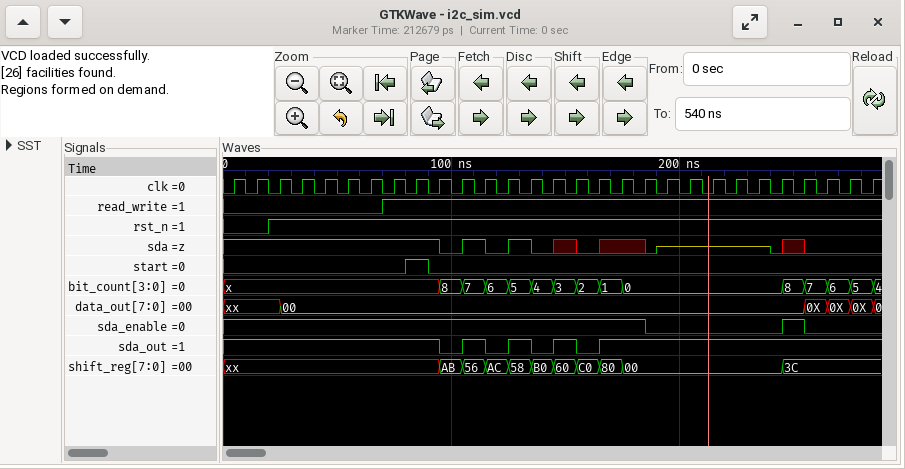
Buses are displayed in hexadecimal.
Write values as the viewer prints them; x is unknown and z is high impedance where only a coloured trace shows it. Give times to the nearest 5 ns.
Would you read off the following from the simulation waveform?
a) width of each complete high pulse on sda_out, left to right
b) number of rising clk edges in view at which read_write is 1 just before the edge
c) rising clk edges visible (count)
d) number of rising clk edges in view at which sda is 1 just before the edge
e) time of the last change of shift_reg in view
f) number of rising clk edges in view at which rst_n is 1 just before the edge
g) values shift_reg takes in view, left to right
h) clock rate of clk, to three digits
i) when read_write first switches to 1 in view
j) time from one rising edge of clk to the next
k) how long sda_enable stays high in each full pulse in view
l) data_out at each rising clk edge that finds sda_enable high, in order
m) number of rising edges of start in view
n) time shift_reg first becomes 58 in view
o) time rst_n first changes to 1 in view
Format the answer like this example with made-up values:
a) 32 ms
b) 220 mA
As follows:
a) 10 ns, 10 ns, 10 ns
b) 22
c) 29
d) 12
e) 245 ns
f) 27
g) xx, AB, 56, AC, 58, B0, 60, C0, 80, 00, 3C
h) 100 MHz
i) 70 ns
j) 10 ns
k) 10 ns
l) xx, xx, xx, 00, 00, 00, 00, 00, 00, 00, 00, 00, 00, 00, 00, 00, 00, 00, 00, 00
m) 1
n) 125 ns
o) 20 ns
